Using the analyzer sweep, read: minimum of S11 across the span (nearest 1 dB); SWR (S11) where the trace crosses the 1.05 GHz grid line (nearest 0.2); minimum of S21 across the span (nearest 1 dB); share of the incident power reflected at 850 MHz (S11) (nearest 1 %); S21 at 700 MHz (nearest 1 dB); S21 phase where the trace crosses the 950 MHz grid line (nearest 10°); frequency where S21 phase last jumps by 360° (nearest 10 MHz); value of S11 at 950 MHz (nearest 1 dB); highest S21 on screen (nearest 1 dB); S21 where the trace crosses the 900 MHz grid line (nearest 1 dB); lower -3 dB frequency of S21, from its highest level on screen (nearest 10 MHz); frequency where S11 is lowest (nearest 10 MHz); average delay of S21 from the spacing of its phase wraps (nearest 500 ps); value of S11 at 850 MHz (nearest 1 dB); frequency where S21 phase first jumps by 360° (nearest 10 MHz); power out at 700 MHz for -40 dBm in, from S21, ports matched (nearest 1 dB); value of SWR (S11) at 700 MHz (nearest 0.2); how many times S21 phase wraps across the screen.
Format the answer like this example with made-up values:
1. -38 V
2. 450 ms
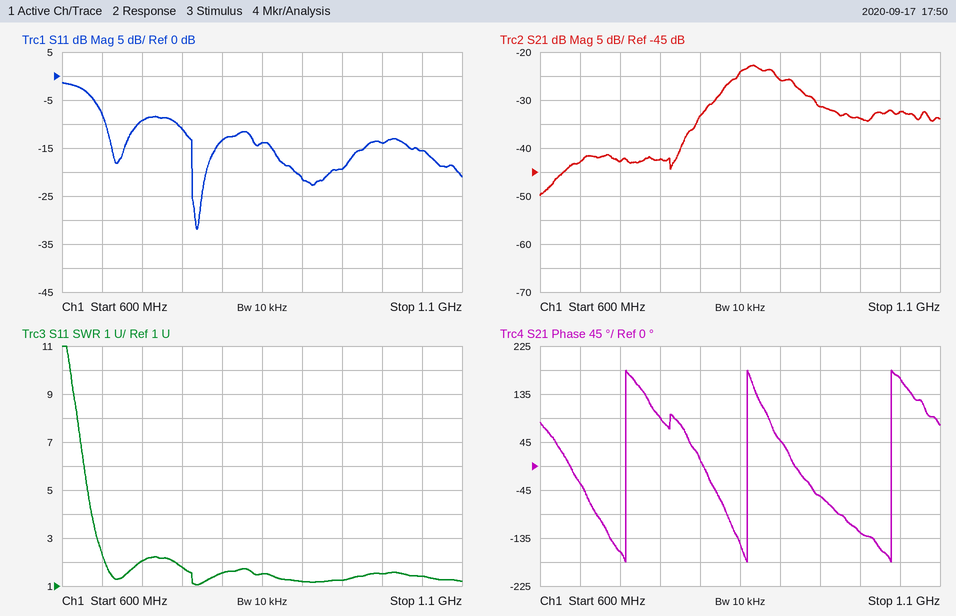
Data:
1. -32 dB
2. 1.4
3. -50 dB
4. 4 %
5. -43 dB
6. -60°
7. 1.04 GHz
8. -19 dB
9. -23 dB
10. -26 dB
11. 840 MHz
12. 770 MHz
13. 6.0 ns
14. -14 dB
15. 710 MHz
16. -83 dBm
17. 2.0
18. 3
